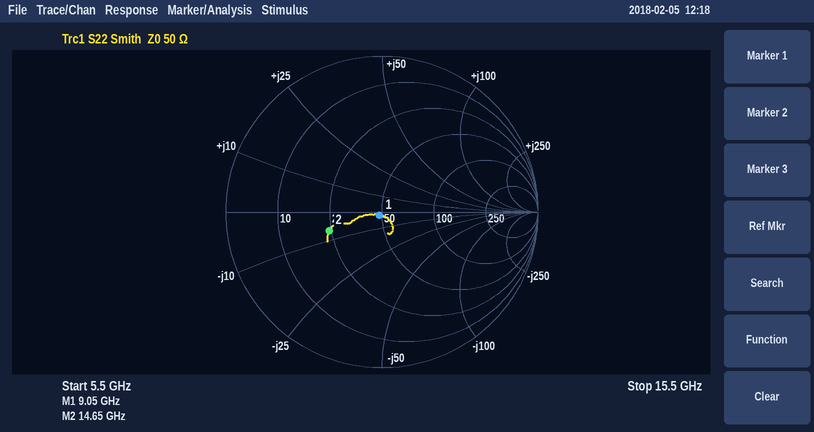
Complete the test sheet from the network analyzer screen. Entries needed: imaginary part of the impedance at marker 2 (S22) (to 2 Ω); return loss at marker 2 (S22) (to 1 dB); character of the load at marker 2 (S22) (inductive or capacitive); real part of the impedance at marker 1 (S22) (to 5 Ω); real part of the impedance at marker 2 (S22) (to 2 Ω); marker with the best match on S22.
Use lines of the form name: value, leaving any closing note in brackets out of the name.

imaginary part of the impedance at marker 2 (S22): -6 Ω
return loss at marker 2 (S22): 9 dB
character of the load at marker 2 (S22): capacitive
real part of the impedance at marker 1 (S22): 50 Ω
real part of the impedance at marker 2 (S22): 24 Ω
marker with the best match on S22: marker 1
